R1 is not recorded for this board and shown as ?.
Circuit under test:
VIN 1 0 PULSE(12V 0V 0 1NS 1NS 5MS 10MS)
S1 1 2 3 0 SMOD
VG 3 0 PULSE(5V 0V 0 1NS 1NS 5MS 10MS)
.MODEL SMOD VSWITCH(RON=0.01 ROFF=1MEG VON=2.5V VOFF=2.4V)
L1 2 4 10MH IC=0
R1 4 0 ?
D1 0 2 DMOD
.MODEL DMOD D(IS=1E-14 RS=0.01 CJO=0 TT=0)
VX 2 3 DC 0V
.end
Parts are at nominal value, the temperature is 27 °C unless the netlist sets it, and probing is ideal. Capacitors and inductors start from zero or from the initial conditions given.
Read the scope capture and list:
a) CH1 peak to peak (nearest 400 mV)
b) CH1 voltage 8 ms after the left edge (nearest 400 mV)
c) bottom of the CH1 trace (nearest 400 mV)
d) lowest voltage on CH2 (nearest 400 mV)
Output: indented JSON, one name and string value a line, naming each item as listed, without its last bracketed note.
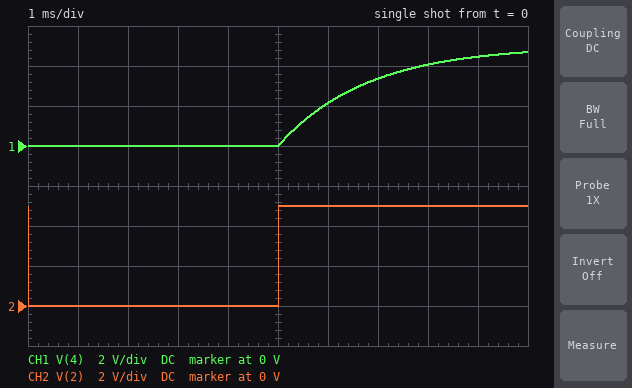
{
  "CH1 peak to peak": "4.8 V",
  "CH1 voltage 8 ms after the left edge": "4.0 V",
  "bottom of the CH1 trace": "0 V",
  "lowest voltage on CH2": "0 V"
}
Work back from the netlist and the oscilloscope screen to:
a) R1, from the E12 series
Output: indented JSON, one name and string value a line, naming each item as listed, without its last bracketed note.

{
  "R1, from the E12 series": "5.6 Ω"
}
